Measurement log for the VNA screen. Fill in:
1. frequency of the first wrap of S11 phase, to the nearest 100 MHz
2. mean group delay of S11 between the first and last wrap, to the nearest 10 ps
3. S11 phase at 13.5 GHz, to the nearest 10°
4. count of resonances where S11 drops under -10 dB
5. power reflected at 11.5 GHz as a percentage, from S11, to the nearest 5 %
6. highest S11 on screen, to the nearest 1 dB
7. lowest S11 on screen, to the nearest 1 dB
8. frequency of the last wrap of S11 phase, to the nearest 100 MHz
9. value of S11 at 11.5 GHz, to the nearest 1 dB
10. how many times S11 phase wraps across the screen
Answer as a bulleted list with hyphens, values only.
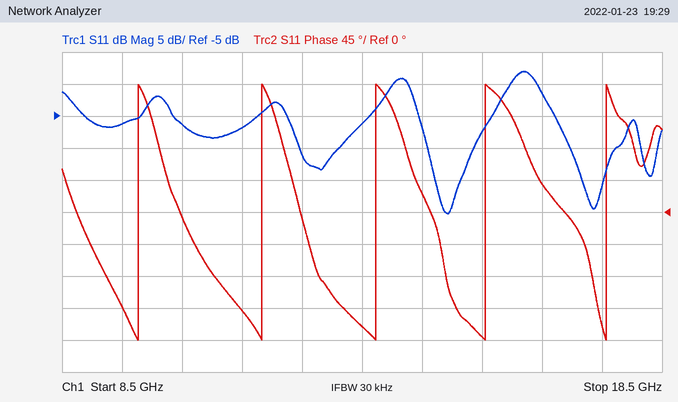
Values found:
- 9.8 GHz
- 510 ps
- -160°
- 4
- 20 %
- 2 dB
- -20 dB
- 17.6 GHz
- -7 dB
- 5
